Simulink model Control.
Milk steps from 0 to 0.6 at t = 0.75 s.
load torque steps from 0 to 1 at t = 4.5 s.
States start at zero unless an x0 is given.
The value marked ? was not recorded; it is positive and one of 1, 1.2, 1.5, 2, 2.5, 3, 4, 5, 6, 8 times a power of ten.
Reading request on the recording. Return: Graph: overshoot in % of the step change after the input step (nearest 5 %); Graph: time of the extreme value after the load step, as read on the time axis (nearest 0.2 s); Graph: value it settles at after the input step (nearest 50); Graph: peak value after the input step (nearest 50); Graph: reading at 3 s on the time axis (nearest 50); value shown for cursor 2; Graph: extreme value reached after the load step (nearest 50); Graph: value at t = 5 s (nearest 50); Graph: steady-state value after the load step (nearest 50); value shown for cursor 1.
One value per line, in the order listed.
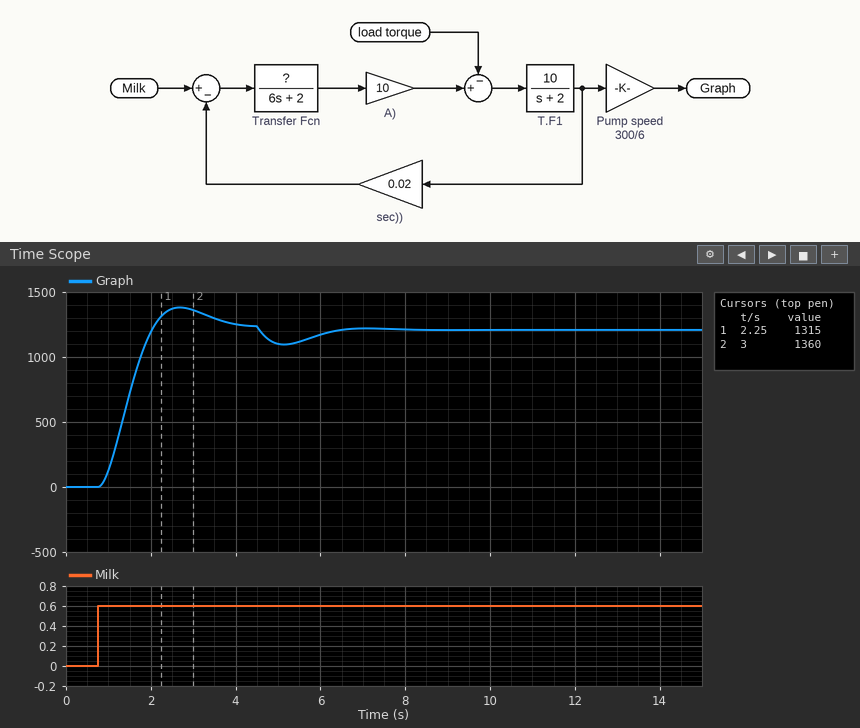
10 %
5.2 s
1250
1400
1350
1360
1100
1100
1200
1315
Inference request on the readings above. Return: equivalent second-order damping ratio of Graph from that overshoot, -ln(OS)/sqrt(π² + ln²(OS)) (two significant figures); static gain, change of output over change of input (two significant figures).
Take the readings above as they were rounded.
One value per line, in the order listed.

0.59
2100
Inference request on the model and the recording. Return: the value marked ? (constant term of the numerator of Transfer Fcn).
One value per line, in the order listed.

10
